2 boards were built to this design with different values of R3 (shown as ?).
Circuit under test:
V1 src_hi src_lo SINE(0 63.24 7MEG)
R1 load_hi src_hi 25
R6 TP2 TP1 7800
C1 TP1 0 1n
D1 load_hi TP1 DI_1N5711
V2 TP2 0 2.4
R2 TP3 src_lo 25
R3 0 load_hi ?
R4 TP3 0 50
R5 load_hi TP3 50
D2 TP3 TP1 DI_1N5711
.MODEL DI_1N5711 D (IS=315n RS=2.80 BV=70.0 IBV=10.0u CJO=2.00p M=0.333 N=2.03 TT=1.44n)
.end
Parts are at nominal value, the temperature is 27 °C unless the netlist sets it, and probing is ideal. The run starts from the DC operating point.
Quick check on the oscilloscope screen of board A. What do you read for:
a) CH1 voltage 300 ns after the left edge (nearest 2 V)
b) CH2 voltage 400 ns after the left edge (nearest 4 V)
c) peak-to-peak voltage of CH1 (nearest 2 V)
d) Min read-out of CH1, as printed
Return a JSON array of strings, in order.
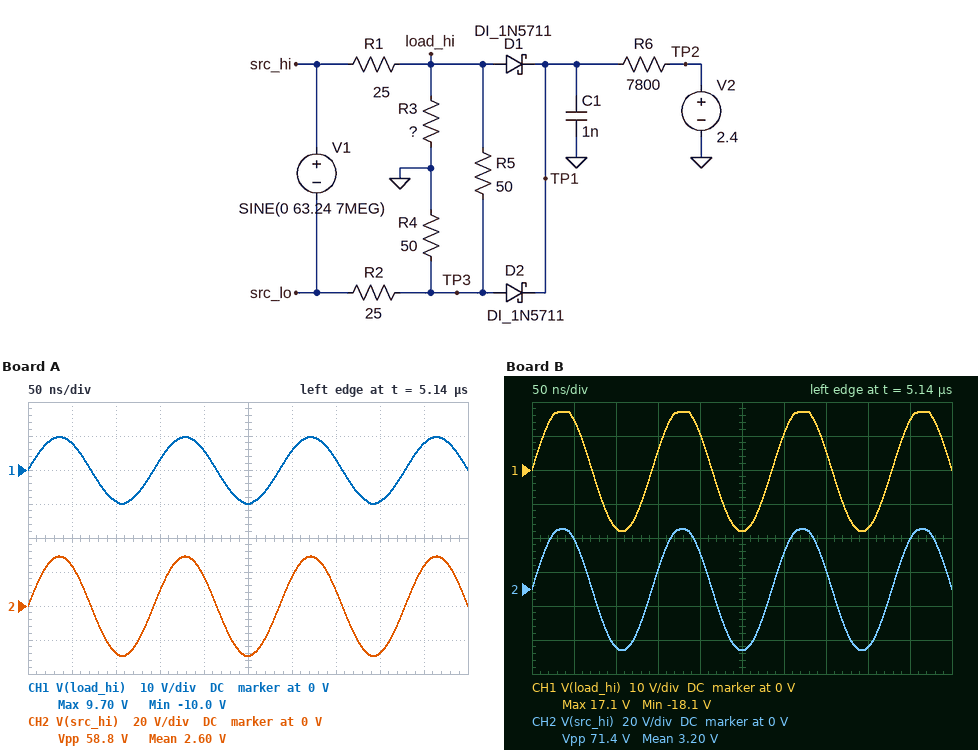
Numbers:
["6 V", "-28 V", "20 V", "-10.0 V"]
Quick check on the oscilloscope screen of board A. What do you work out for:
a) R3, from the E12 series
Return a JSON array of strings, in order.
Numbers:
["33 Ω"]
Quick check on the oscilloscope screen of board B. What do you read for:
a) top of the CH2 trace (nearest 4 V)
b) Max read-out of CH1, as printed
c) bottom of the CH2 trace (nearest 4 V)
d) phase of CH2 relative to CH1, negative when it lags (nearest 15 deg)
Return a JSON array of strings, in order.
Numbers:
["36 V", "17.1 V", "-36 V", "0 deg"]
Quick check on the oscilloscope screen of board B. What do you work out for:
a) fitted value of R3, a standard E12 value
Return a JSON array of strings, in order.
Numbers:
["100 Ω"]
